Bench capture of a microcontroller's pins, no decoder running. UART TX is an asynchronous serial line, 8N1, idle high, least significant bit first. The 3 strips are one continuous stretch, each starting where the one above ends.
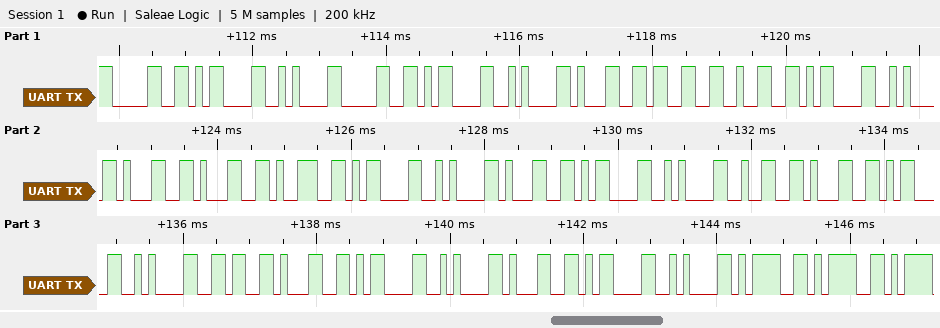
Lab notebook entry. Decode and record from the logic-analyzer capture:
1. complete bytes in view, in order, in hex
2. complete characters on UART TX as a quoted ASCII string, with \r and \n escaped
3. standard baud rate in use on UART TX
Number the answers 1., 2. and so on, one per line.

1. 0x30 0x0D 0x0A 0x30 0x0D 0x0A 0x31 0x33 0x32 0x0D 0x0A 0x31 0x31 0x39 0x0D 0x0A 0x31 0x0D 0x0A 0x32 0x31 0x0D 0x0A 0x36 0x31 0x0D 0x0A 0x31 0x0D 0x0A 0x3D 0x3D
2. "0\r\n0\r\n132\r\n119\r\n1\r\n21\r\n61\r\n1\r\n=="
3. 9600 baud
